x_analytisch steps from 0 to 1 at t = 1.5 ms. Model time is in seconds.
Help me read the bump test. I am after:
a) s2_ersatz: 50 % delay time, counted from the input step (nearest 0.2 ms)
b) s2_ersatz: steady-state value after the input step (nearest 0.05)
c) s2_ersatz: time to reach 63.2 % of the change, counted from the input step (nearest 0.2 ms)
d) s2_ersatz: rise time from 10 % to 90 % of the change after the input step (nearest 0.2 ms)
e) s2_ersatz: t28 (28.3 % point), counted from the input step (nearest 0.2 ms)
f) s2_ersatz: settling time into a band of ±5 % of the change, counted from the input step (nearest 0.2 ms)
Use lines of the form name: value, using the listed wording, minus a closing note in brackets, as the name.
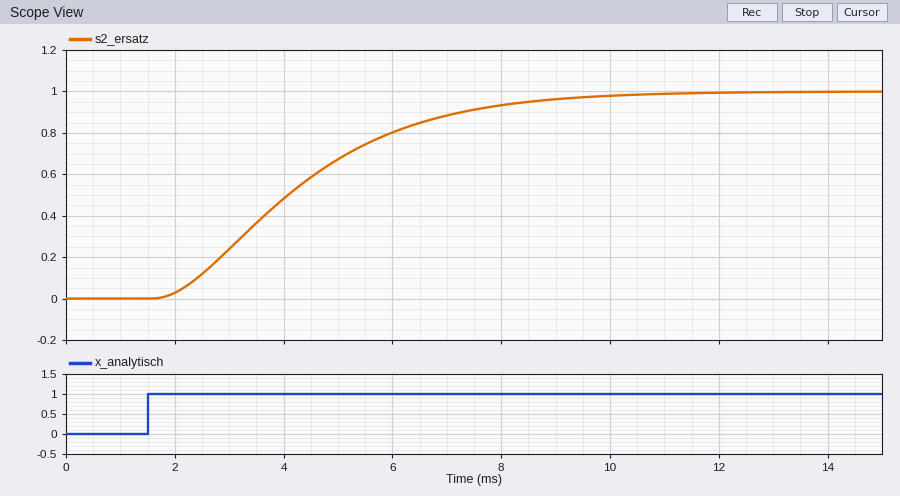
s2_ersatz: 50 % delay time, counted from the input step: 2.6 ms
s2_ersatz: steady-state value after the input step: 1.00
s2_ersatz: time to reach 63.2 % of the change, counted from the input step: 3.2 ms
s2_ersatz: rise time from 10 % to 90 % of the change after the input step: 4.8 ms
s2_ersatz: t28 (28.3 % point), counted from the input step: 1.6 ms
s2_ersatz: settling time into a band of ±5 % of the change, counted from the input step: 7.0 ms
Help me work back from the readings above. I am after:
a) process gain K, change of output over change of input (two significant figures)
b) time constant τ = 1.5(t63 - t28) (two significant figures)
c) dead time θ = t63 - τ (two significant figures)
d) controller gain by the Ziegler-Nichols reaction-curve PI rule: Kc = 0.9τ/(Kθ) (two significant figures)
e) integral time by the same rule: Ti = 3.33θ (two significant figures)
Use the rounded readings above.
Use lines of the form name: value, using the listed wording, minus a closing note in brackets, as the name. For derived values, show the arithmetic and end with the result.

process gain K, change of output over change of input: (1 - 0) / 1 = 1.0
time constant τ = 1.5(t63 - t28): 1.5 × (3.2 - 1.6) = 2.4 ms
dead time θ = t63 - τ: 3.2 - 2.4 = 0.80 ms
controller gain by the Ziegler-Nichols reaction-curve PI rule: Kc = 0.9τ/(Kθ): 0.9 × 2.4 / (1 × 0.8) = 2.7
integral time by the same rule: Ti = 3.33θ: 3.33 × 0.8 = 2.7 ms
